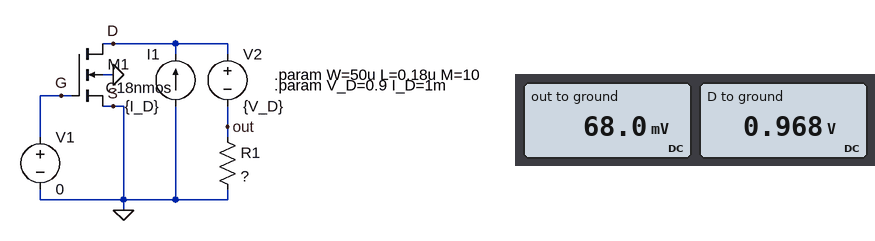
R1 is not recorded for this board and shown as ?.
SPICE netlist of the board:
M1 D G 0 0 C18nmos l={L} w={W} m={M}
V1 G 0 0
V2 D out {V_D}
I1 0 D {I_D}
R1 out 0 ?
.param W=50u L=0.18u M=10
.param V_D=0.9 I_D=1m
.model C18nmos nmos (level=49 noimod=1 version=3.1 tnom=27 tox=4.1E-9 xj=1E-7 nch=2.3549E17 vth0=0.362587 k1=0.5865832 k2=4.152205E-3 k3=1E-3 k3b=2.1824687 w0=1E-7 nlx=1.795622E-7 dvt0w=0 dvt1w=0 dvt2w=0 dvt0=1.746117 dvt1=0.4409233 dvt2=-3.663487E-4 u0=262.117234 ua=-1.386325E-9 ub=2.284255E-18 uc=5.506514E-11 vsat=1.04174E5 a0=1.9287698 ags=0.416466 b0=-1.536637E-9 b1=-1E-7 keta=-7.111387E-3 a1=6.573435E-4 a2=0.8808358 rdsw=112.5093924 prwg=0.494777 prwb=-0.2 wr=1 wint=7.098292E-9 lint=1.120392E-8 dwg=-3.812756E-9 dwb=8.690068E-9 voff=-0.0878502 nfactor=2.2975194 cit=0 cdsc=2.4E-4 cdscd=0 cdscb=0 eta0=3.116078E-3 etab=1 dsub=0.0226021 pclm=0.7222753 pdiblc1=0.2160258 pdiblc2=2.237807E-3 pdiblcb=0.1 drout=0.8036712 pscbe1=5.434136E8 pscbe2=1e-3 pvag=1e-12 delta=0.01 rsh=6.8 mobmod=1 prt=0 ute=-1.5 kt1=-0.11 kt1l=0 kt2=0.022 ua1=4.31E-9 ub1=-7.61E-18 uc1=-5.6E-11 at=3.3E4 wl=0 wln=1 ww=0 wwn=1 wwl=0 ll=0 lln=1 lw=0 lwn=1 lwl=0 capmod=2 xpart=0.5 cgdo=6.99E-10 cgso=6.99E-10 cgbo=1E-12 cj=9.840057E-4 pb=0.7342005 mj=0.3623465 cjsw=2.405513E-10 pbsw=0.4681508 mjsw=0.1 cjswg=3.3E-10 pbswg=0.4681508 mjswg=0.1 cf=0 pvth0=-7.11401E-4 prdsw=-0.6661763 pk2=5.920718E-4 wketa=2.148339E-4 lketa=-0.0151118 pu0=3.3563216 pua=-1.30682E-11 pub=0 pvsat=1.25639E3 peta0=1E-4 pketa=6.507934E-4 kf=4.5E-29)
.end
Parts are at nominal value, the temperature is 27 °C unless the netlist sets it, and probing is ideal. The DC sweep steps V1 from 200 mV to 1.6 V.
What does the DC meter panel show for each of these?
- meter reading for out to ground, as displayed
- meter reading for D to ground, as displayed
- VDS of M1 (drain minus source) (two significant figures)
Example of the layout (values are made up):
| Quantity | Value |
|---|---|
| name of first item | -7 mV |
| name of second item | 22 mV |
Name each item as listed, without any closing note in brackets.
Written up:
| Quantity | Value |
|---|---|
| meter reading for out to ground, as displayed | 68.0 mV |
| meter reading for D to ground, as displayed | 0.968 V |
| VDS of M1 (drain minus source) | 970 mV |
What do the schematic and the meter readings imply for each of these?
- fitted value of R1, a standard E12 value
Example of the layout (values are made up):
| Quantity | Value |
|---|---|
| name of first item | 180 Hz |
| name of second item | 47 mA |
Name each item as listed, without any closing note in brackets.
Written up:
| Quantity | Value |
|---|---|
| fitted value of R1, a standard E12 value | 68 Ω |
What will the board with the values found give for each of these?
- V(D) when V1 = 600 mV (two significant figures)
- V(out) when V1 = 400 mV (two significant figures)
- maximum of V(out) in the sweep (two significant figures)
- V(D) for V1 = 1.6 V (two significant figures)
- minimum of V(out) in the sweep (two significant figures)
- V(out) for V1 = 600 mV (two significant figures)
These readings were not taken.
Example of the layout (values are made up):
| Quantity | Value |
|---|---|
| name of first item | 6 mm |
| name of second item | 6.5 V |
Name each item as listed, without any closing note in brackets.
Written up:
| Quantity | Value |
|---|---|
| V(D) when V1 = 600 mV | 600 mV |
| V(out) when V1 = 400 mV | 59 mV |
| maximum of V(out) in the sweep | 68 mV |
| V(D) for V1 = 1.6 V | 40 mV |
| minimum of V(out) in the sweep | -860 mV |
| V(out) for V1 = 600 mV | -300 mV |
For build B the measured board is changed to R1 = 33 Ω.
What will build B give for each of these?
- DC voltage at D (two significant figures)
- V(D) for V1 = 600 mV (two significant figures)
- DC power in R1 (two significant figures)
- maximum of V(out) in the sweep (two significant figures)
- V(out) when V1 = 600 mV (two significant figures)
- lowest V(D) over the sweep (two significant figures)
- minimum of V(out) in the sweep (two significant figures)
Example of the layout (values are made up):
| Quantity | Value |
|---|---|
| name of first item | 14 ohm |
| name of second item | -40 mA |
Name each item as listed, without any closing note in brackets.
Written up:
| Quantity | Value |
|---|---|
| DC voltage at D | 930 mV |
| V(D) for V1 = 600 mV | 750 mV |
| DC power in R1 | 33 µW |
| maximum of V(out) in the sweep | 33 mV |
| V(out) when V1 = 600 mV | -150 mV |
| lowest V(D) over the sweep | 77 mV |
| minimum of V(out) in the sweep | -820 mV |
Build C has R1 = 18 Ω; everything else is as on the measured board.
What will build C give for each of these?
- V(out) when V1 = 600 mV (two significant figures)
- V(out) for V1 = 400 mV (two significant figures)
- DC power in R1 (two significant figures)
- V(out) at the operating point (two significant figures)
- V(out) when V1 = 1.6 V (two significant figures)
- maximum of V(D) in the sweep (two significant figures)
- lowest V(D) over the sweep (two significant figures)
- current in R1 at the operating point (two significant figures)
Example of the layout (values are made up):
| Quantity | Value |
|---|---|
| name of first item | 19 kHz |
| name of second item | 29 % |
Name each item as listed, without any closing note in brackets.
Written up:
| Quantity | Value |
|---|---|
| V(out) when V1 = 600 mV | -85 mV |
| V(out) for V1 = 400 mV | 16 mV |
| DC power in R1 | 18 µW |
| V(out) at the operating point | 18 mV |
| V(out) when V1 = 1.6 V | -770 mV |
| maximum of V(D) in the sweep | 920 mV |
| lowest V(D) over the sweep | 130 mV |
| current in R1 at the operating point | 1.0 mA |
